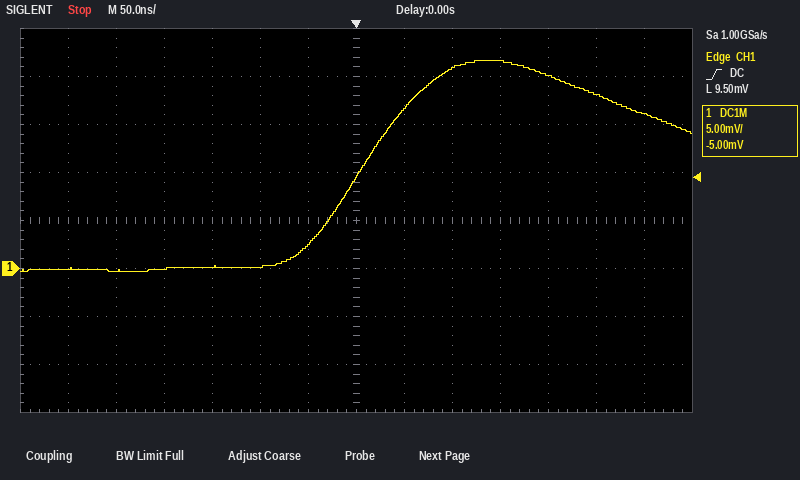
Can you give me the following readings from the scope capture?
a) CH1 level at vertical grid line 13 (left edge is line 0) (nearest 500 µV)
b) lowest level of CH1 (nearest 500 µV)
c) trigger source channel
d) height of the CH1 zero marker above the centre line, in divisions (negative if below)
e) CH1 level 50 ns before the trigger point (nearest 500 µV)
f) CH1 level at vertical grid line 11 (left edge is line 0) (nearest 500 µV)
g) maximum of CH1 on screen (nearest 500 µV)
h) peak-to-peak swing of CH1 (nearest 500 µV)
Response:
16.0 mV
-500 µV
CH1
-1.0 div
2.5 mV
20.0 mV
21.5 mV
22.0 mV
